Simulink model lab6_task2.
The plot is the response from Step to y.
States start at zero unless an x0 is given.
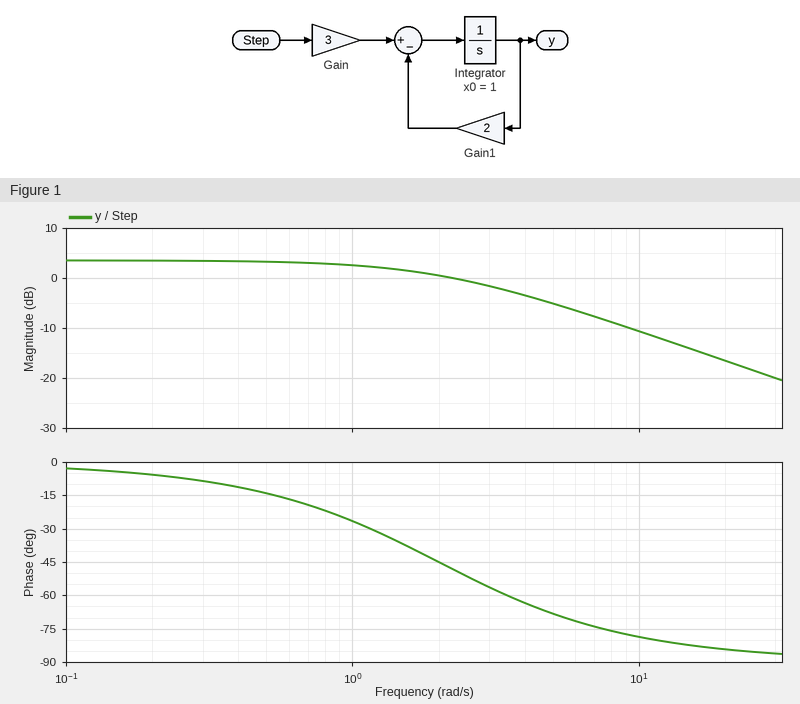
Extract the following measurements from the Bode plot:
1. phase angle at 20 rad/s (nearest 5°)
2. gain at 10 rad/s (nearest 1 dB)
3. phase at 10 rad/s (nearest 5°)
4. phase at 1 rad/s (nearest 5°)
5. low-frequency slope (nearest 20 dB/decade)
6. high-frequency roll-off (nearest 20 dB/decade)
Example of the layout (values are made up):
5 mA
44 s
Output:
-85°
-11 dB
-80°
-25°
0 dB/decade
-20 dB/decade
